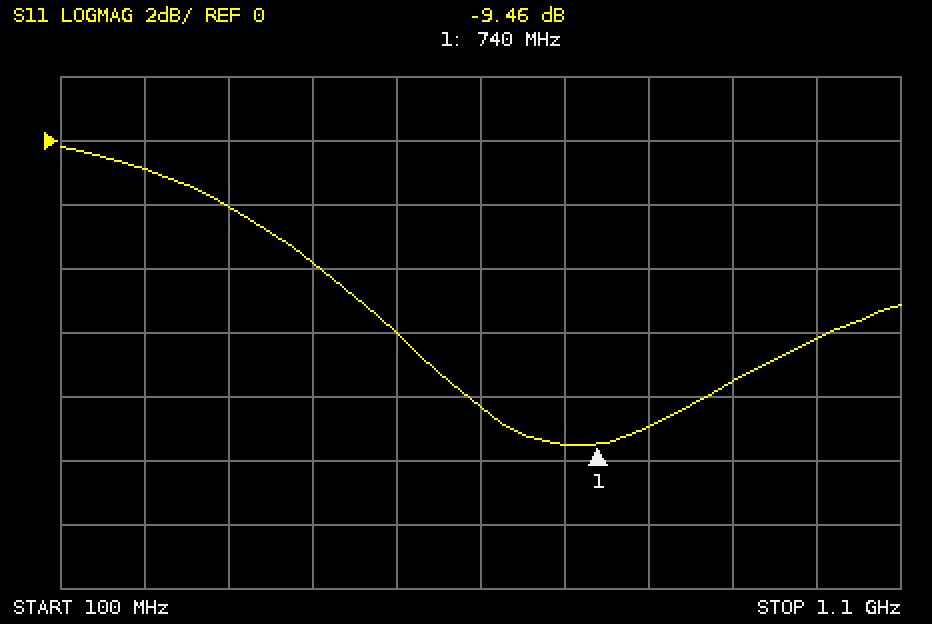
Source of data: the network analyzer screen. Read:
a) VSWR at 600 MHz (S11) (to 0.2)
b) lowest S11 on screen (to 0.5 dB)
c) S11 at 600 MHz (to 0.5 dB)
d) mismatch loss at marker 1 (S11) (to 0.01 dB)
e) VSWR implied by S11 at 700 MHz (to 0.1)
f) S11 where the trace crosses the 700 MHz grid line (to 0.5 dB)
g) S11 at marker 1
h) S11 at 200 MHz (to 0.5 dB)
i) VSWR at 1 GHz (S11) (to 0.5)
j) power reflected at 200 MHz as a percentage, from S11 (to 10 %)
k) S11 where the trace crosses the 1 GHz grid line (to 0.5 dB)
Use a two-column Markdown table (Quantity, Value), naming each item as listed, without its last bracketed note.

| Quantity | Value |
|---|---|
| VSWR at 600 MHz (S11) | 2.2 |
| lowest S11 on screen | -9.5 dB |
| S11 at 600 MHz | -8.5 dB |
| mismatch loss at marker 1 (S11) | 0.52 dB |
| VSWR implied by S11 at 700 MHz | 2.0 |
| S11 where the trace crosses the 700 MHz grid line | -9.5 dB |
| S11 at marker 1 | -9.46 dB |
| S11 at 200 MHz | -1.0 dB |
| VSWR at 1 GHz (S11) | 3.0 |
| power reflected at 200 MHz as a percentage, from S11 | 80 % |
| S11 where the trace crosses the 1 GHz grid line | -6.0 dB |
